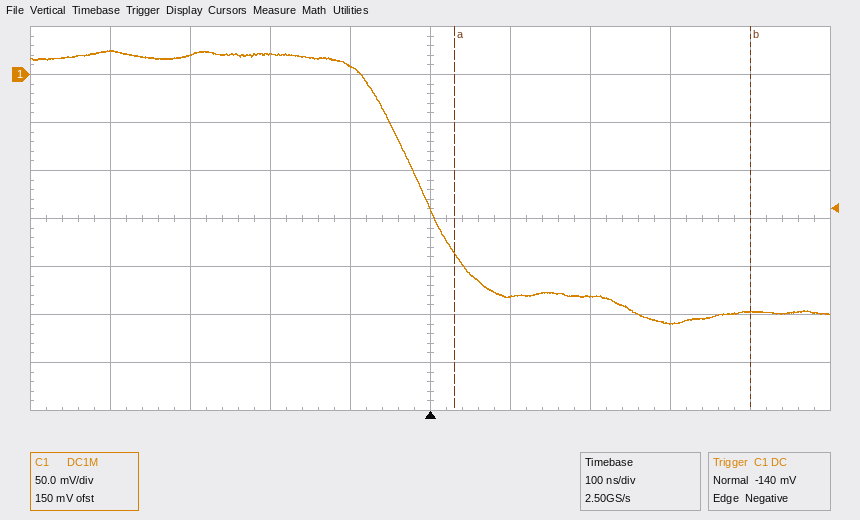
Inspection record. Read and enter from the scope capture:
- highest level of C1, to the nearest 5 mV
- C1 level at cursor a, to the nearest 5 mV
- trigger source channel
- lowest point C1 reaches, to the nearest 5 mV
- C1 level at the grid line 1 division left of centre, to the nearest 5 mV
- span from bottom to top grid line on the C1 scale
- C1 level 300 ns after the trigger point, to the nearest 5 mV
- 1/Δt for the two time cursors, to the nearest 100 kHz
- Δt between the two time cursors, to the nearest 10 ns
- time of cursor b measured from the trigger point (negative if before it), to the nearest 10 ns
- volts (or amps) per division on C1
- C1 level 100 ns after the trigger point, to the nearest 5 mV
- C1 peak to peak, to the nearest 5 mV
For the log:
25 mV
-185 mV
C1
-260 mV
10 mV
400 mV
-260 mV
2.7 MHz
370 ns
+400 ns
50 mV
-230 mV
285 mV
